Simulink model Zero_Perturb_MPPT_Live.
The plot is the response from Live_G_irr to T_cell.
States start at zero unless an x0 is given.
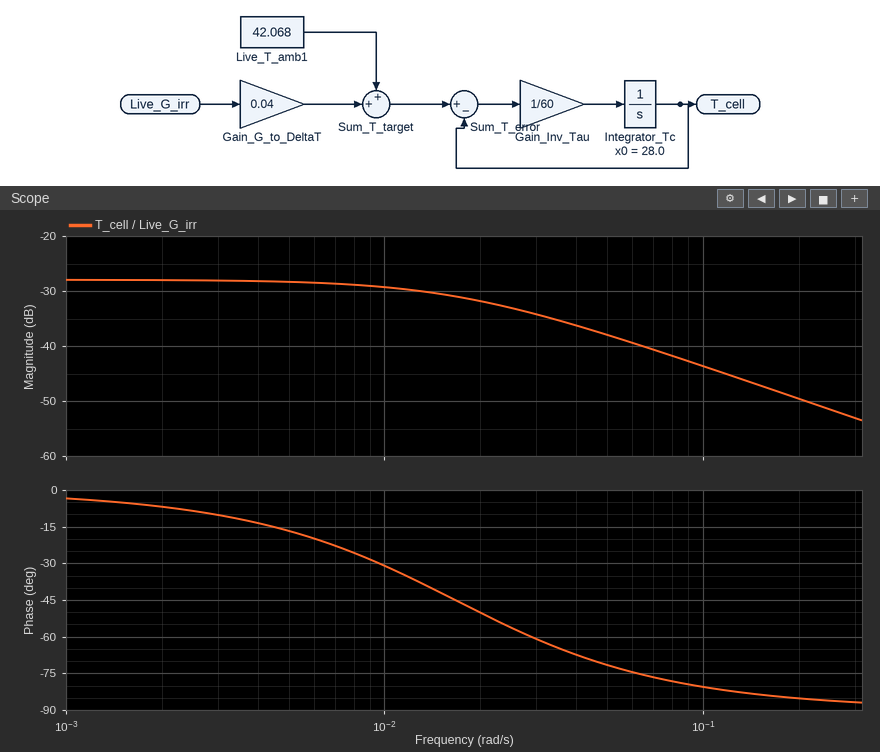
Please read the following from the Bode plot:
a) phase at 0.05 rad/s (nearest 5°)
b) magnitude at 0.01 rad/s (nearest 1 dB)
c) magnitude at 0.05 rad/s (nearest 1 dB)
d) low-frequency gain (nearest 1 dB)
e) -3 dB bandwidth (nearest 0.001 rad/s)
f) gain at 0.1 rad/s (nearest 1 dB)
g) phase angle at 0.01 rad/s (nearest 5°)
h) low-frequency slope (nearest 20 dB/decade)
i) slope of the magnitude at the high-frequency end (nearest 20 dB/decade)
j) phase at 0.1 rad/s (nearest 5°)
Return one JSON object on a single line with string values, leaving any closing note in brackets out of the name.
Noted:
{"phase at 0.05 rad/s": "-70°", "magnitude at 0.01 rad/s": "-29 dB", "magnitude at 0.05 rad/s": "-38 dB", "low-frequency gain": "-28 dB", "-3 dB bandwidth": "0.017 rad/s", "gain at 0.1 rad/s": "-44 dB", "phase angle at 0.01 rad/s": "-30°", "low-frequency slope": "0 dB/decade", "slope of the magnitude at the high-frequency end": "-20 dB/decade", "phase at 0.1 rad/s": "-80°"}
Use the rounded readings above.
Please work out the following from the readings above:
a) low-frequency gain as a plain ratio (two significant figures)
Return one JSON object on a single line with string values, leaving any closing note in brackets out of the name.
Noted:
{"low-frequency gain as a plain ratio": "0.040"}
